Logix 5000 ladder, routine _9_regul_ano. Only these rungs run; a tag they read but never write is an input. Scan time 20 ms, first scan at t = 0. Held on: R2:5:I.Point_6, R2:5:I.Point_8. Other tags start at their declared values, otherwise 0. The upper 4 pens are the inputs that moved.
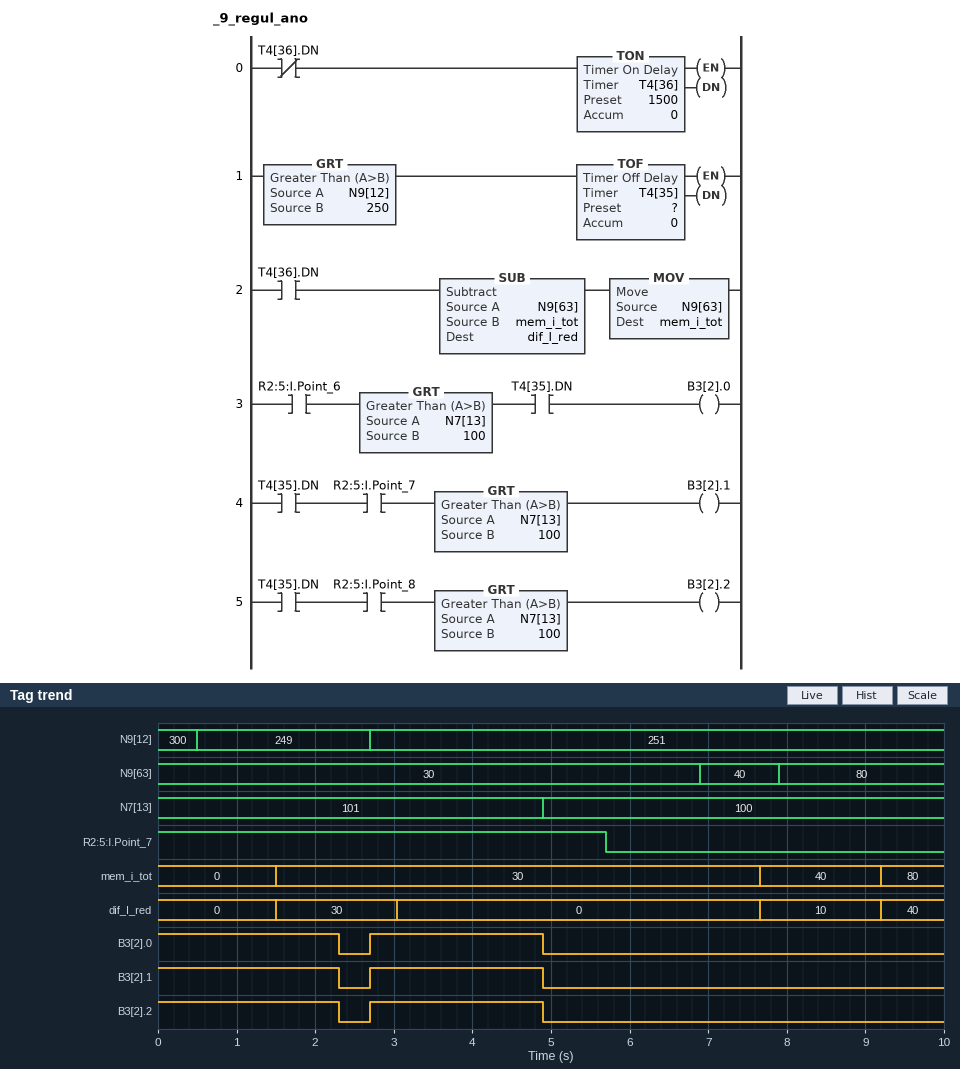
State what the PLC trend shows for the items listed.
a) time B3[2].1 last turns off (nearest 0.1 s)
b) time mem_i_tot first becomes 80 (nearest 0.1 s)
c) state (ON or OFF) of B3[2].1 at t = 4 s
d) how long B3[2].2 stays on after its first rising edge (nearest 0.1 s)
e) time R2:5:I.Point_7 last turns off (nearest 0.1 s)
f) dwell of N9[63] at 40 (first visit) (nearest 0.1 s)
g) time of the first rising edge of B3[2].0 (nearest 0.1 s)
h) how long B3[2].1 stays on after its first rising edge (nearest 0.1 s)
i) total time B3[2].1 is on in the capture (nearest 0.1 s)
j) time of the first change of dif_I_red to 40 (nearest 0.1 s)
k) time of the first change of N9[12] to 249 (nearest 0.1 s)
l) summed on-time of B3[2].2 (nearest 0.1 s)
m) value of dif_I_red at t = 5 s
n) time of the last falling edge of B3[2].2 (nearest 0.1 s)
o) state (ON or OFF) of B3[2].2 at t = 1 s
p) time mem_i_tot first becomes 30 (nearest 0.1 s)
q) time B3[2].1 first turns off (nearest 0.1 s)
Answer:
4.9 s
9.2 s
ON
2.2 s
5.7 s
1.0 s
2.7 s
2.2 s
4.5 s
9.2 s
0.5 s
4.5 s
0
4.9 s
ON
1.5 s
2.3 s
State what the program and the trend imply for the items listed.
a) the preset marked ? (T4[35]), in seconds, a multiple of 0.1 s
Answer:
1.8 s
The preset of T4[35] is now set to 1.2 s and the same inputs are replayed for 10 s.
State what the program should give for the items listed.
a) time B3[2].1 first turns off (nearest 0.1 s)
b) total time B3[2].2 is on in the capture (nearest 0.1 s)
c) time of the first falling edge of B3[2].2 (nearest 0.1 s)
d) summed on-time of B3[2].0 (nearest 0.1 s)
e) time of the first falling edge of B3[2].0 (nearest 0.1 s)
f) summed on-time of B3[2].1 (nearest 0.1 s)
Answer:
1.7 s
3.9 s
1.7 s
3.9 s
1.7 s
3.9 s
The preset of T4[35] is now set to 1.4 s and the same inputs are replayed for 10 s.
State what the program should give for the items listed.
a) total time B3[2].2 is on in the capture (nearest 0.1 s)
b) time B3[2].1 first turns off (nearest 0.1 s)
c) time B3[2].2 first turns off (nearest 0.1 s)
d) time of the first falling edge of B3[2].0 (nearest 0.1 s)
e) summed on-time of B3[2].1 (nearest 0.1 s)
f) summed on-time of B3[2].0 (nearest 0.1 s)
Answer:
4.1 s
1.9 s
1.9 s
1.9 s
4.1 s
4.1 s
